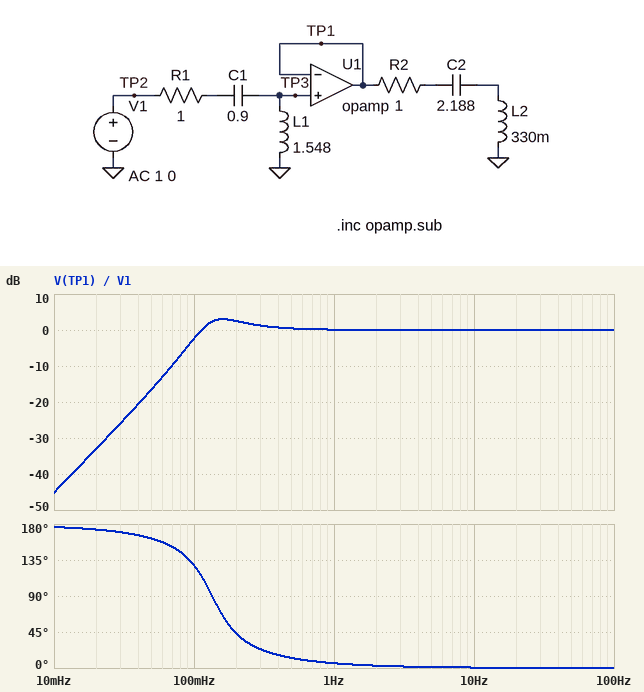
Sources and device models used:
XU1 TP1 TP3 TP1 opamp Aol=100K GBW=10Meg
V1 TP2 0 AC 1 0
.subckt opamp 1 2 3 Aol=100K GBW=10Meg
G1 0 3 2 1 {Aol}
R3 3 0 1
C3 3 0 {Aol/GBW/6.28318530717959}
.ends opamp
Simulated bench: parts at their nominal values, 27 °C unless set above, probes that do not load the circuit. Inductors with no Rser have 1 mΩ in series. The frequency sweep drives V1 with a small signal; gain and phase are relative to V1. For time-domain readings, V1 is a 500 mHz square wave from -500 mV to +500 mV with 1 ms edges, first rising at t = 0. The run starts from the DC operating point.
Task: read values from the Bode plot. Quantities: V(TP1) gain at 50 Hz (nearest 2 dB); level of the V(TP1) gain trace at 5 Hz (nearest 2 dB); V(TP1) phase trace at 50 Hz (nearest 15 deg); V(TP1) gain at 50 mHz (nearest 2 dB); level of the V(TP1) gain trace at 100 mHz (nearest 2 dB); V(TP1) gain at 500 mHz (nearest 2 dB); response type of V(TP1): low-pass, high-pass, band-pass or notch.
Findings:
0 dB
0 dB
0 deg
-16 dB
-2 dB
0 dB
high-pass
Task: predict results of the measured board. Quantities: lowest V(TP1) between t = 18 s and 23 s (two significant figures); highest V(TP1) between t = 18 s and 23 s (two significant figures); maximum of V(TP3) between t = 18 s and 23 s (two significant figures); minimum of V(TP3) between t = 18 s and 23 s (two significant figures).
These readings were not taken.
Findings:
-680 mV
680 mV
680 mV
-680 mV
